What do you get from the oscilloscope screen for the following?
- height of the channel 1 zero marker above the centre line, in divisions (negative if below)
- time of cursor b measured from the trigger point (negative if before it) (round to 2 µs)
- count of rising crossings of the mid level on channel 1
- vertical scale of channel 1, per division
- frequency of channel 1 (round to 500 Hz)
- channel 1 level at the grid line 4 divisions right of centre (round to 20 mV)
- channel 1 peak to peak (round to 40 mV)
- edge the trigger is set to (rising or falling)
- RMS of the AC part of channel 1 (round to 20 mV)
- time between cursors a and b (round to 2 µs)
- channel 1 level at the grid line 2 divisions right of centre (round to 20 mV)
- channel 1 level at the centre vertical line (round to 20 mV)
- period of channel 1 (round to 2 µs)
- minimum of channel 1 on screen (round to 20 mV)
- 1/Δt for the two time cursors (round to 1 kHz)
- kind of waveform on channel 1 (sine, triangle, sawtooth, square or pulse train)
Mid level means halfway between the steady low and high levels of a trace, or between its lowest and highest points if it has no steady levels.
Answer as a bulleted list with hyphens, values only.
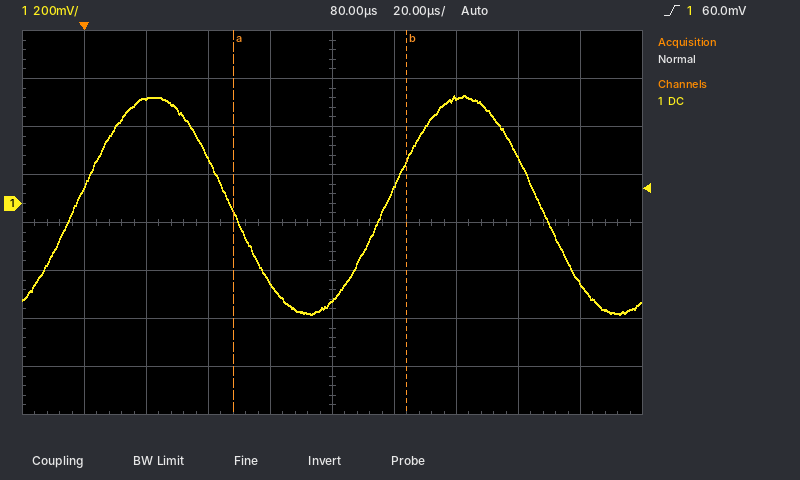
- +0.4 div
- +104 µs
- 2
- 200 mV
- 10.0 kHz
- -340 mV
- 920 mV
- rising
- 320 mV
- 56 µs
- 440 mV
- -400 mV
- 100 µs
- -460 mV
- 18 kHz
- sine
